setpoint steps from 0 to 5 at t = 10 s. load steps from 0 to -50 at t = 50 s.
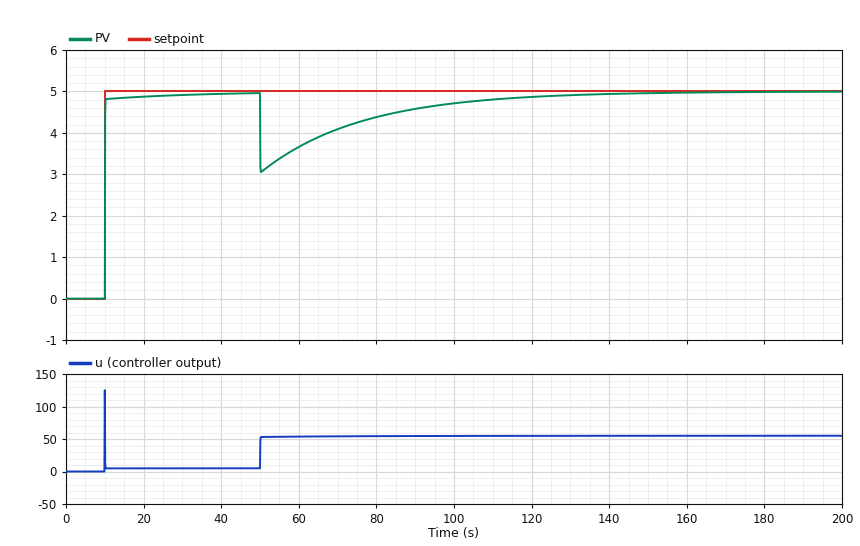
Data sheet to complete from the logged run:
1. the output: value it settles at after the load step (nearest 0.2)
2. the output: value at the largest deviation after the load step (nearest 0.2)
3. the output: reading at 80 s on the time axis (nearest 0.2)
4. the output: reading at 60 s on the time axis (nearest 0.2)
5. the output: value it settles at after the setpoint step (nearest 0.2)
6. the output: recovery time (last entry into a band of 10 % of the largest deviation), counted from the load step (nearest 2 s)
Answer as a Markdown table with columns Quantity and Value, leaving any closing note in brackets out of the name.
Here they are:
| Quantity | Value |
|---|---|
| the output: value it settles at after the load step | 5.0 |
| the output: value at the largest deviation after the load step | 3.0 |
| the output: reading at 80 s on the time axis | 4.4 |
| the output: reading at 60 s on the time axis | 3.6 |
| the output: value it settles at after the setpoint step | 5.0 |
| the output: recovery time (last entry into a band of 10 % of the largest deviation), counted from the load step | 60 s |
